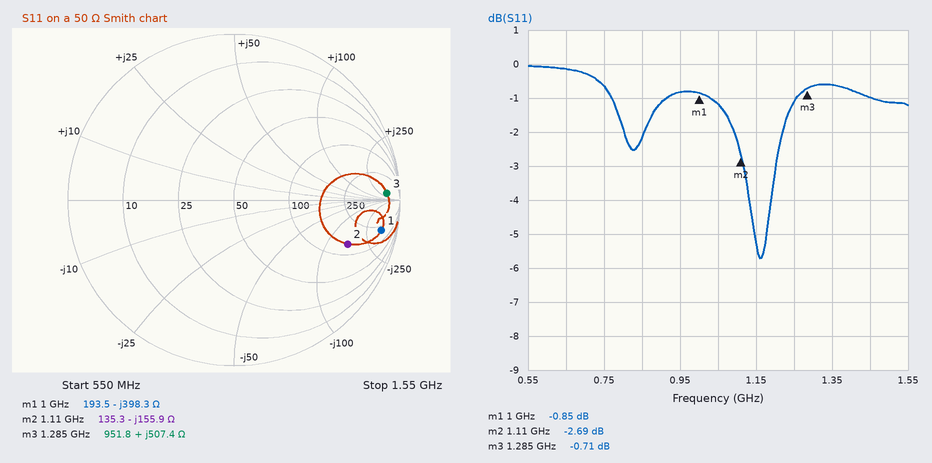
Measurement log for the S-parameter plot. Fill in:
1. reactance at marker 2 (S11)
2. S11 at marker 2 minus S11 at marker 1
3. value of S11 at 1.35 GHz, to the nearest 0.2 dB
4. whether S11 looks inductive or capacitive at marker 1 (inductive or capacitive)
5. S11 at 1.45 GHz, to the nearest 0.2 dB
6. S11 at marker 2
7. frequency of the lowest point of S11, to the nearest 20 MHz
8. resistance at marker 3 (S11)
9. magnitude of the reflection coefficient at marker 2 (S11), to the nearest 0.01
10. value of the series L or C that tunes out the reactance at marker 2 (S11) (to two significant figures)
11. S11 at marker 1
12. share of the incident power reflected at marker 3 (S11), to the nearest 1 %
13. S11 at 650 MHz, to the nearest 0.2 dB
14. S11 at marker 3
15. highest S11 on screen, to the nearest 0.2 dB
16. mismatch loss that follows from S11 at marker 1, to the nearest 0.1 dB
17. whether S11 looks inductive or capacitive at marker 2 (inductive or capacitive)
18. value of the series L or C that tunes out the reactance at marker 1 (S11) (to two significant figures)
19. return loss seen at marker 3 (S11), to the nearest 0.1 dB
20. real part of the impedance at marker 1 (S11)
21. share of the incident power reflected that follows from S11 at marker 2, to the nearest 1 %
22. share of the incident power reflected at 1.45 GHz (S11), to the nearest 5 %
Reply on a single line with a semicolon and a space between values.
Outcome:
-155.9 Ω; -1.84 dB; -0.6 dB; capacitive; -1.0 dB; -2.69 dB; 1.16 GHz; 951.8 Ω; 0.73; 22 nH; -0.85 dB; 85 %; -0.2 dB; -0.71 dB; 0.0 dB; 7.5 dB; capacitive; 63 nH; 0.7 dB; 193.5 Ω; 54 %; 80 %
